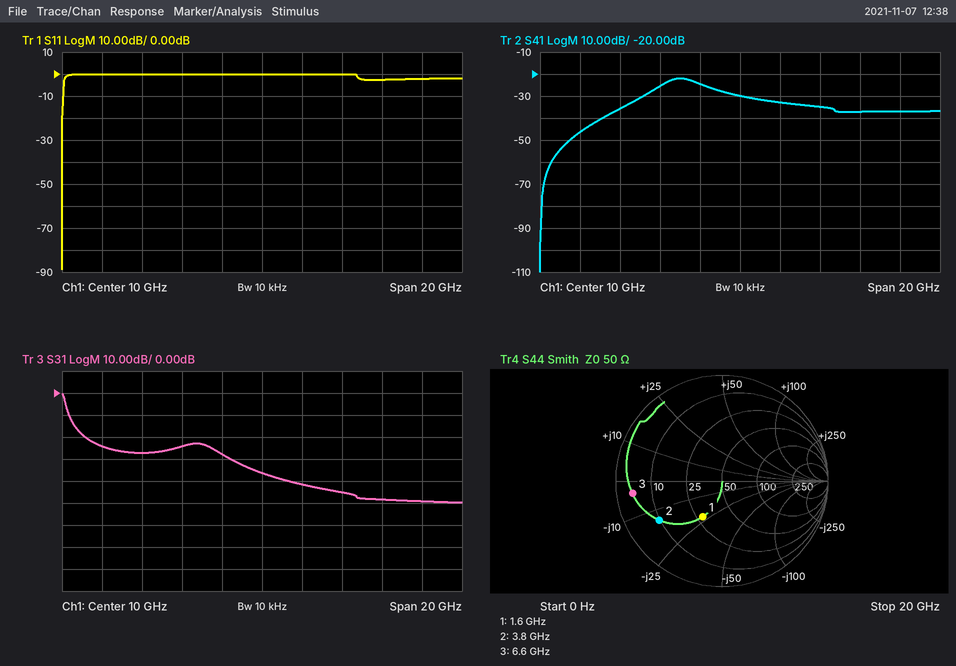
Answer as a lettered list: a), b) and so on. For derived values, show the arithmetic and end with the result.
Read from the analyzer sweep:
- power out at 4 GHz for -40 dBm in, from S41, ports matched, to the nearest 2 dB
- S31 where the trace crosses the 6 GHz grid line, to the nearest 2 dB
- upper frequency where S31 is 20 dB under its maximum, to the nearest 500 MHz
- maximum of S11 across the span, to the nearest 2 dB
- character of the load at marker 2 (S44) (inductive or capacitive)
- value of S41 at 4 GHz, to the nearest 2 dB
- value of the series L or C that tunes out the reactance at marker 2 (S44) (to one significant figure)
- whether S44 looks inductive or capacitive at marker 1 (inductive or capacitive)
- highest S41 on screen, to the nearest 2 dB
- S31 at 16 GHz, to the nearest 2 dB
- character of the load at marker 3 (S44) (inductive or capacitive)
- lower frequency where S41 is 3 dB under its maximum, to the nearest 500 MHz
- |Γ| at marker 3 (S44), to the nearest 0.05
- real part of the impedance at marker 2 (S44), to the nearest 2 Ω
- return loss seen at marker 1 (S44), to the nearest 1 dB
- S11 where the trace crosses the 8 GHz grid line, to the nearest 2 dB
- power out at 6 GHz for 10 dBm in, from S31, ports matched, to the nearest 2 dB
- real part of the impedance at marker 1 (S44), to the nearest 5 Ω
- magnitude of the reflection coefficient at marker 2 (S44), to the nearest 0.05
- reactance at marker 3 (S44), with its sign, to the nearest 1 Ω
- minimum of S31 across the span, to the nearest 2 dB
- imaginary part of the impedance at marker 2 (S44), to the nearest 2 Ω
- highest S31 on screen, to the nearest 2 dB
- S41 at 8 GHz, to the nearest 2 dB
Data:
a) -40 dBm + (-36 dB) = -76 dBm
b) -24 dB
c) 1.0 GHz
d) 0 dB
e) capacitive
f) -36 dB
g) L = 14 Ω/(2π × 3.8 GHz) ≈ 586 pH, so 600 pH to one significant figure
h) capacitive
i) -22 dB
j) -48 dB
k) capacitive
l) 6.0 GHz
m) 0.85
n) 10 Ω
o) 8 dB
p) 0 dB
q) 10 dBm + (-24 dB) = -14 dBm
r) 30 Ω
s) 0.70
t) -3 Ω
u) -50 dB
v) -14 Ω
w) 0 dB
x) -24 dB
